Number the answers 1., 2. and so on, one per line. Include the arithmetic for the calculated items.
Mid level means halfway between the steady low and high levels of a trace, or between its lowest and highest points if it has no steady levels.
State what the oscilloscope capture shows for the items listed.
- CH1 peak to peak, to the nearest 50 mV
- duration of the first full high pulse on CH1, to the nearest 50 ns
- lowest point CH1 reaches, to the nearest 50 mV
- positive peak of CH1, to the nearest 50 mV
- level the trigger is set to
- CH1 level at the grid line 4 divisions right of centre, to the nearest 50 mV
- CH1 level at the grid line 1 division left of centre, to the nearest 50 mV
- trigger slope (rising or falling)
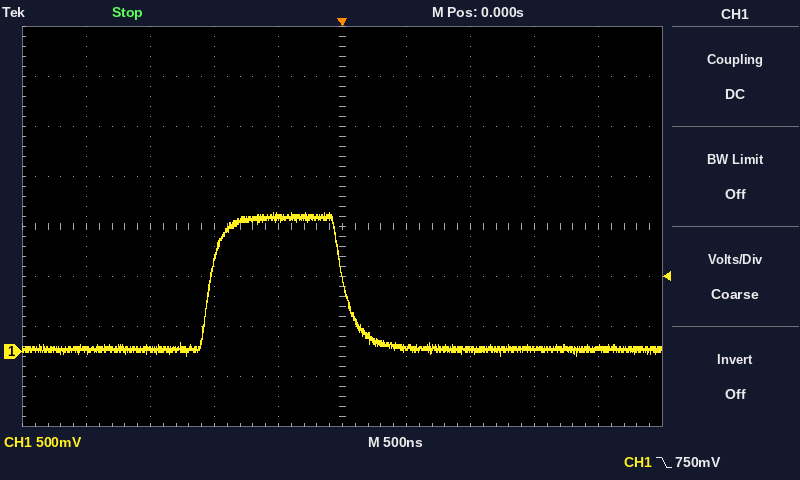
1. 1.40 V − (-50 mV) = 1.45 V
2. 1.05 µs
3. -50 mV
4. 1.40 V
5. 750 mV
6. 50 mV
7. 1.35 V
8. falling
